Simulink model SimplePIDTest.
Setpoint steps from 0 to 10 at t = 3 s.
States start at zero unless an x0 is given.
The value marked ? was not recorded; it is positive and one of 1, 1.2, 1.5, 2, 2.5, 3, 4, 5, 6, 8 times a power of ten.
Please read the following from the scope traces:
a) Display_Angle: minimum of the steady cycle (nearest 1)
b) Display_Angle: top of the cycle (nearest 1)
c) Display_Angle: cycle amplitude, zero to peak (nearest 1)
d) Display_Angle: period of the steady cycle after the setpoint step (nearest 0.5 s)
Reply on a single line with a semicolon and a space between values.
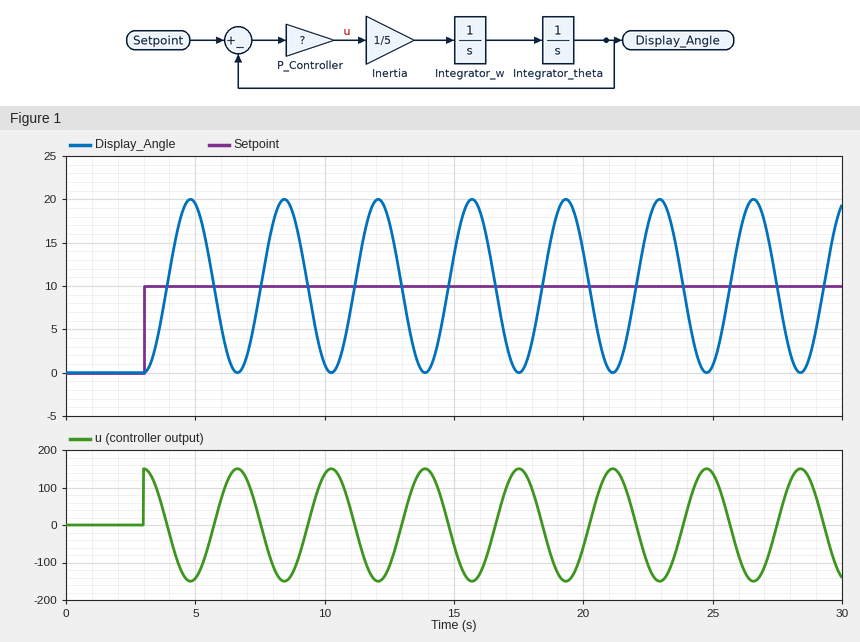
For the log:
0; 20; 10; 3.5 s
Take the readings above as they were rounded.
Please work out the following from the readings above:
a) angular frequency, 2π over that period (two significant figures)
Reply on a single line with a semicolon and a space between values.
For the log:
1.8 rad/s
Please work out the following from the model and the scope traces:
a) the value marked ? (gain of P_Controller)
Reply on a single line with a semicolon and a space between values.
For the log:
15
